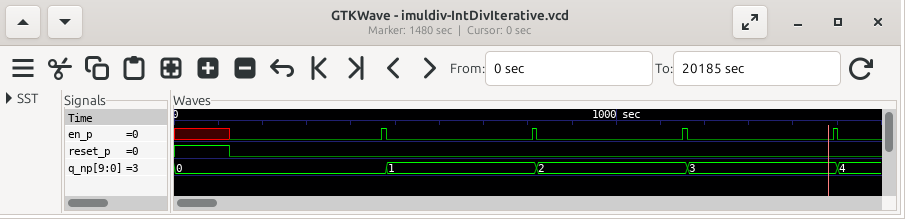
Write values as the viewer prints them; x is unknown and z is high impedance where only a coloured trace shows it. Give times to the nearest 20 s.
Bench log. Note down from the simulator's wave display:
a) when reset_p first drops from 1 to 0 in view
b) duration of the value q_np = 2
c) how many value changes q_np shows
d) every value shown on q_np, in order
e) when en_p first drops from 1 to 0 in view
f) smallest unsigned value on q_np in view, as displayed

120 s
340 s
4
0, 1, 2, 3, 4
480 s
0
